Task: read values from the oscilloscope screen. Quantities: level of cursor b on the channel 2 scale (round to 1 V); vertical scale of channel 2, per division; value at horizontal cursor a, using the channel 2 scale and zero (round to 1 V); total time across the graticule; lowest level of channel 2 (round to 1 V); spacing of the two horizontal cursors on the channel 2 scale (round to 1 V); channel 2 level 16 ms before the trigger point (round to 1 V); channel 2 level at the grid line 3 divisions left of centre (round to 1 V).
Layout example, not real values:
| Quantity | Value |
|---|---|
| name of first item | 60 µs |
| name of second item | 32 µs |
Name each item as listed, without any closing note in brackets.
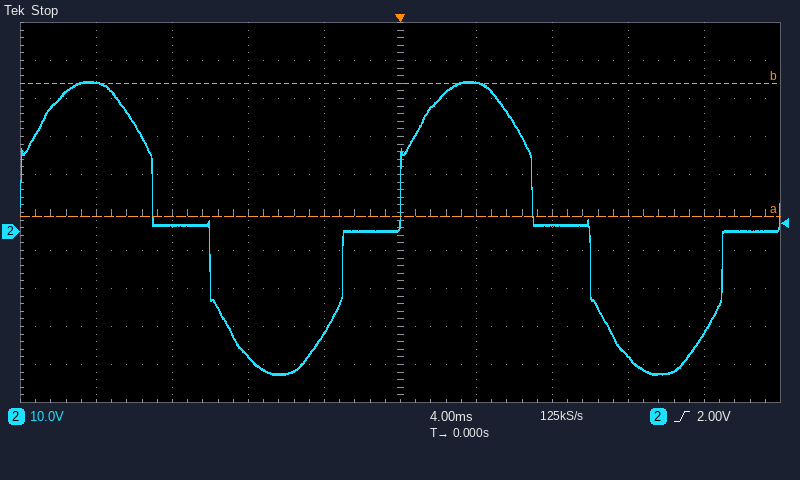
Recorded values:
| Quantity | Value |
|---|---|
| level of cursor b on the channel 2 scale | 39 V |
| vertical scale of channel 2, per division | 10 V |
| value at horizontal cursor a, using the channel 2 scale and zero | 4 V |
| total time across the graticule | 40 ms |
| lowest level of channel 2 | -38 V |
| spacing of the two horizontal cursors on the channel 2 scale | 35 V |
| channel 2 level 16 ms before the trigger point | 39 V |
| channel 2 level at the grid line 3 divisions left of centre | 2 V |
